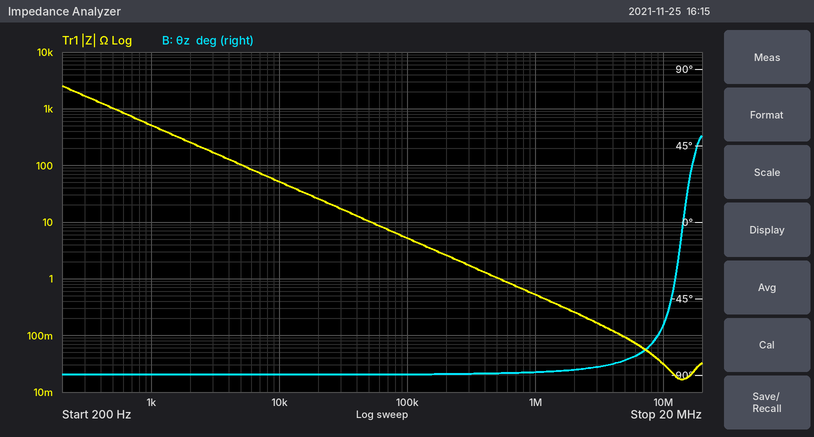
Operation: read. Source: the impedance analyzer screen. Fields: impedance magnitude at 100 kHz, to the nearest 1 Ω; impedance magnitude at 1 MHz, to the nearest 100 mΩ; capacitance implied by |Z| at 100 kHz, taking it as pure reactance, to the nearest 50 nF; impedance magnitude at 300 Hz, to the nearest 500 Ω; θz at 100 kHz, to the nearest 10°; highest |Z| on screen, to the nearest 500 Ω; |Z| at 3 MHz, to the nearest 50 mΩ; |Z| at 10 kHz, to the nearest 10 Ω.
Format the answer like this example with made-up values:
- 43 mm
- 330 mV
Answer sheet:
- 5 Ω
- 500 mΩ
- 300 nF
- 1.5 kΩ
- -90°
- 2.5 kΩ
- 150 mΩ
- 50 Ω
